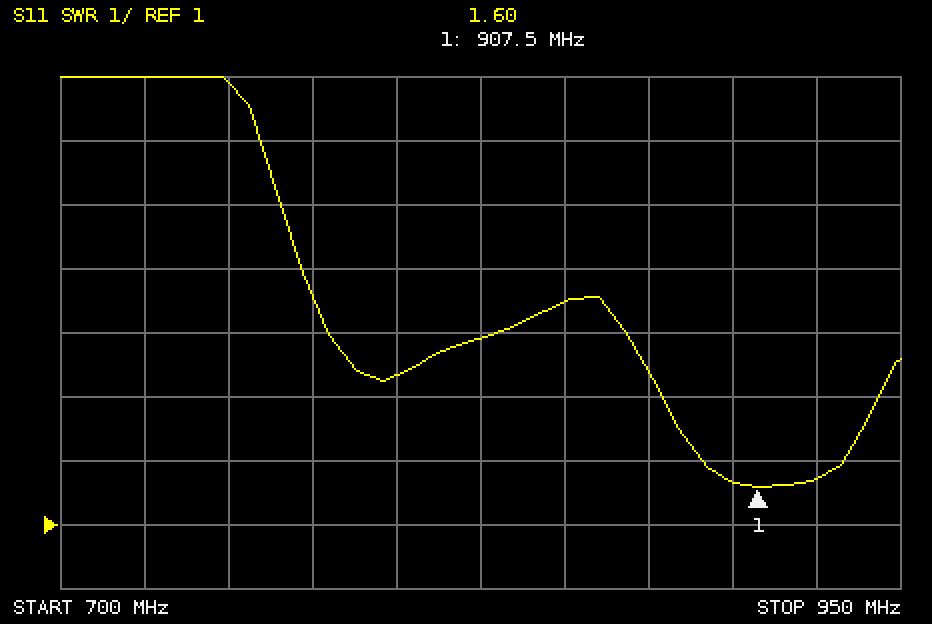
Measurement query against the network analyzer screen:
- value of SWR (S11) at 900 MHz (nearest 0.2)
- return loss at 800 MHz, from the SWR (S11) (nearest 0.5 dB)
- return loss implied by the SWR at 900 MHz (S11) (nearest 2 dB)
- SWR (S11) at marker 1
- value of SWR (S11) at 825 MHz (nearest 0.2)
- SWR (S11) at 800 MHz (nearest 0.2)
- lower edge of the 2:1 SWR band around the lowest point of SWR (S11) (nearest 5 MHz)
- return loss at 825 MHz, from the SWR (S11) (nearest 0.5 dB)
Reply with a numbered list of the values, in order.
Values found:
1. 1.6
2. 5.5 dB
3. 12 dB
4. 1.60
5. 4.0
6. 3.4
7. 890 MHz
8. 4.5 dB
